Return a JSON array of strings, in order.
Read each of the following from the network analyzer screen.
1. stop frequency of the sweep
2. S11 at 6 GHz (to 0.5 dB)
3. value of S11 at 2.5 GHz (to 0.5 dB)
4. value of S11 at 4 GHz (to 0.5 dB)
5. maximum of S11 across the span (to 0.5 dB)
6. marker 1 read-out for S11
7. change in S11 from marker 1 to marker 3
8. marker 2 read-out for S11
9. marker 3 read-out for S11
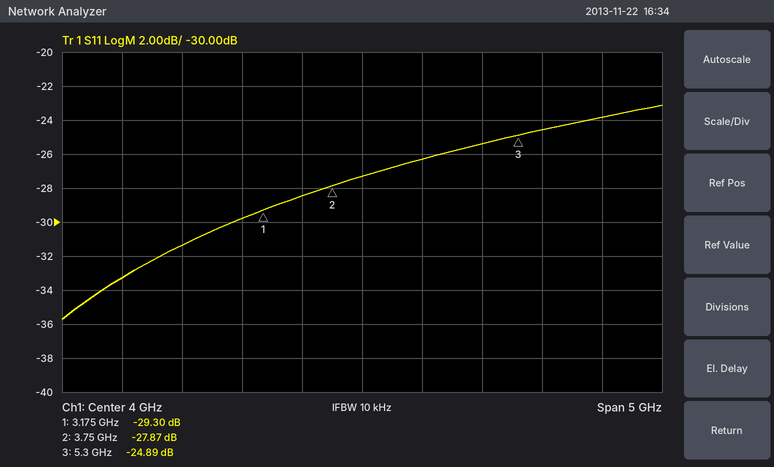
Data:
["6.5 GHz", "-24.0 dB", "-31.5 dB", "-27.5 dB", "-23.0 dB", "-29.30 dB", "4.41 dB", "-27.87 dB", "-24.89 dB"]
